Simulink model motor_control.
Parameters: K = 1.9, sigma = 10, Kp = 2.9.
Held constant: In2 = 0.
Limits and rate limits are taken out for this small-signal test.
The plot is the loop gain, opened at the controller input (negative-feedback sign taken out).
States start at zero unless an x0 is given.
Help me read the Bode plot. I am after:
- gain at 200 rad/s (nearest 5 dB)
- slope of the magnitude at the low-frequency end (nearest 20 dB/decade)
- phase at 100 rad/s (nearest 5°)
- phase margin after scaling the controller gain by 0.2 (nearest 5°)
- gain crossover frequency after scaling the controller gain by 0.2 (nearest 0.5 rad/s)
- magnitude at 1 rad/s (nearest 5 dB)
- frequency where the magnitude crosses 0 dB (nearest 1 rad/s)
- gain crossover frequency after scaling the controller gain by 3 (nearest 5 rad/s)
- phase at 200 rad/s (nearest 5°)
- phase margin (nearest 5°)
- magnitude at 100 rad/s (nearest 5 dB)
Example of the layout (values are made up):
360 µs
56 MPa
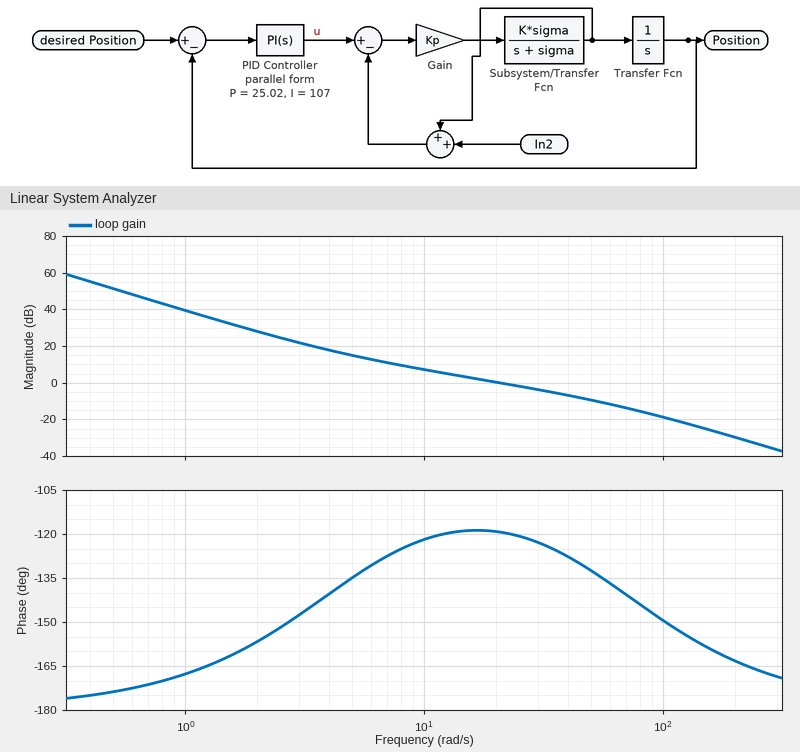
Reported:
-30 dB
-40 dB/decade
-150°
45°
5.5 rad/s
40 dB
21 rad/s
50 rad/s
-165°
60°
-20 dB
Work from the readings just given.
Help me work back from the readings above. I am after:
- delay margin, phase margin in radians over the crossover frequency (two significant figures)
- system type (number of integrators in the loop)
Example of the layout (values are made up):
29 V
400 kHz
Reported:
0.050 s
2
